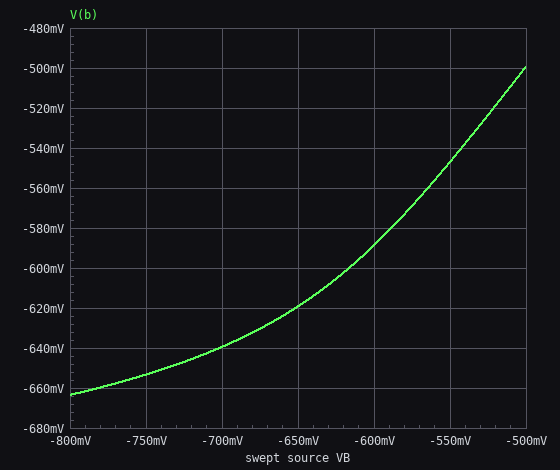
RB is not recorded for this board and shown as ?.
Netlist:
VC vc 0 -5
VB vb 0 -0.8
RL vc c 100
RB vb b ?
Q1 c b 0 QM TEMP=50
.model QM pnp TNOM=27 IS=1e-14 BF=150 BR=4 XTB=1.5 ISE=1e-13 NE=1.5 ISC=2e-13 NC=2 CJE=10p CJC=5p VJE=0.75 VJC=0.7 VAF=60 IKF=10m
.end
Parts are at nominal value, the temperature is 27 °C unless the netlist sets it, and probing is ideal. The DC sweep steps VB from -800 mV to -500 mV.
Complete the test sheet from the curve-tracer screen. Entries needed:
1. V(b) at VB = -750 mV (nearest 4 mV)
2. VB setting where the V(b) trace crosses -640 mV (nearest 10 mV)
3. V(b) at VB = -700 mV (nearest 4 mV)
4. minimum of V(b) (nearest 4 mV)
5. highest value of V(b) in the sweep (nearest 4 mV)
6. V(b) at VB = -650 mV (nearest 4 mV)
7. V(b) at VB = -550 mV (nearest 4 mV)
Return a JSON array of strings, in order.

["-652 mV", "-700 mV", "-640 mV", "-664 mV", "-500 mV", "-620 mV", "-548 mV"]
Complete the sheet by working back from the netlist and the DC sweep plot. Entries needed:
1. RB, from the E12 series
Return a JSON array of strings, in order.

["3.3 kΩ"]
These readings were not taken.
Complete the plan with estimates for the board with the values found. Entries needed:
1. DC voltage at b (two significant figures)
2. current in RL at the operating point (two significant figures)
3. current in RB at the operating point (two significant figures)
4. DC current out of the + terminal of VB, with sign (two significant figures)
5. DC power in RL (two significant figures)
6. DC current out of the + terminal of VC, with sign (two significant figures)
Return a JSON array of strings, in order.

["-660 mV", "4.4 mA", "41 µA", "-41 µA", "2.0 mW", "-4.4 mA"]
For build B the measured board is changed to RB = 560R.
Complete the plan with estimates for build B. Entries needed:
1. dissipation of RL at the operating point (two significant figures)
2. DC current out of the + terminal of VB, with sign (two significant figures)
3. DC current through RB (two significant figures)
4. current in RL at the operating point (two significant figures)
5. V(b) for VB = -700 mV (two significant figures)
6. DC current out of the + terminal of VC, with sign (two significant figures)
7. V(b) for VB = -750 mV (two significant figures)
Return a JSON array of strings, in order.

["15 mW", "-170 µA", "170 µA", "12 mA", "-670 mV", "-12 mA", "-690 mV"]
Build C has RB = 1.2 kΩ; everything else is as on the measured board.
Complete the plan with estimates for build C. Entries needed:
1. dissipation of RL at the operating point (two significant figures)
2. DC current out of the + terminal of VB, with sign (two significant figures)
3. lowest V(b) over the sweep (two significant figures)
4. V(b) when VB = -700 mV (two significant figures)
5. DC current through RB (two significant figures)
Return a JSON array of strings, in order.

["6.8 mW", "-94 µA", "-690 mV", "-660 mV", "94 µA"]
